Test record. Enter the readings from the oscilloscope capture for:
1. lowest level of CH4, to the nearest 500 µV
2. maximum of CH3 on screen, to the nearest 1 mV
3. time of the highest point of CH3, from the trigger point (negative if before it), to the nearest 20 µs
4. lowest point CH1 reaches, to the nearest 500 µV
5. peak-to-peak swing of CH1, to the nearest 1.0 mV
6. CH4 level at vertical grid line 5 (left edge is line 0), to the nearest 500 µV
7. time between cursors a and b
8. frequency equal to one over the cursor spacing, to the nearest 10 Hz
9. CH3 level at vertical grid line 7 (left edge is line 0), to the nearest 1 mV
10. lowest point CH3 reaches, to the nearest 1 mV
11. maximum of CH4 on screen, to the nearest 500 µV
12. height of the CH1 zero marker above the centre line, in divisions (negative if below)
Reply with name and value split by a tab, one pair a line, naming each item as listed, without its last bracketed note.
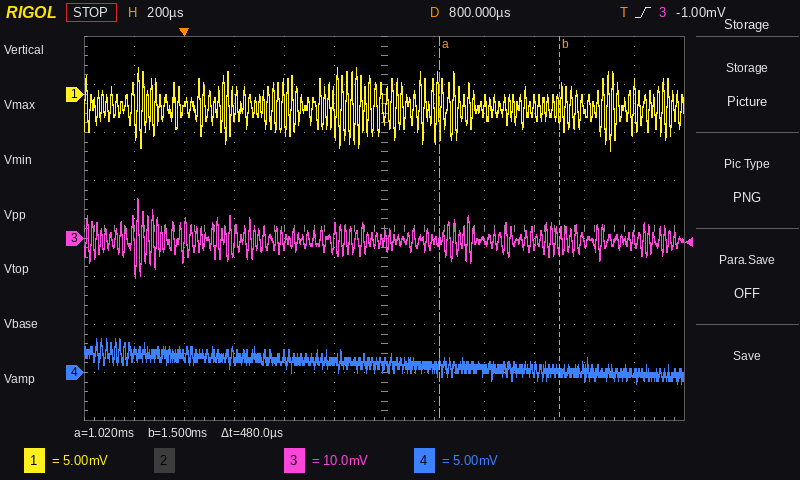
lowest level of CH4, to the nearest 500 µV	-1.0 mV
maximum of CH3 on screen, to the nearest 1 mV	8 mV
time of the highest point of CH3, from the trigger point (negative if before it), to the nearest 20 µs	-180 µs
lowest point CH1 reaches, to the nearest 500 µV	-6.0 mV
peak-to-peak swing of CH1, to the nearest 1.0 mV	9.0 mV
CH4 level at vertical grid line 5 (left edge is line 0), to the nearest 500 µV	1.0 mV
time between cursors a and b	480 µs
frequency equal to one over the cursor spacing, to the nearest 10 Hz	2.08 kHz
CH3 level at vertical grid line 7 (left edge is line 0), to the nearest 1 mV	0 mV
lowest point CH3 reaches, to the nearest 1 mV	-8 mV
maximum of CH4 on screen, to the nearest 500 µV	3.5 mV
height of the CH1 zero marker above the centre line, in divisions	+2.8 div
